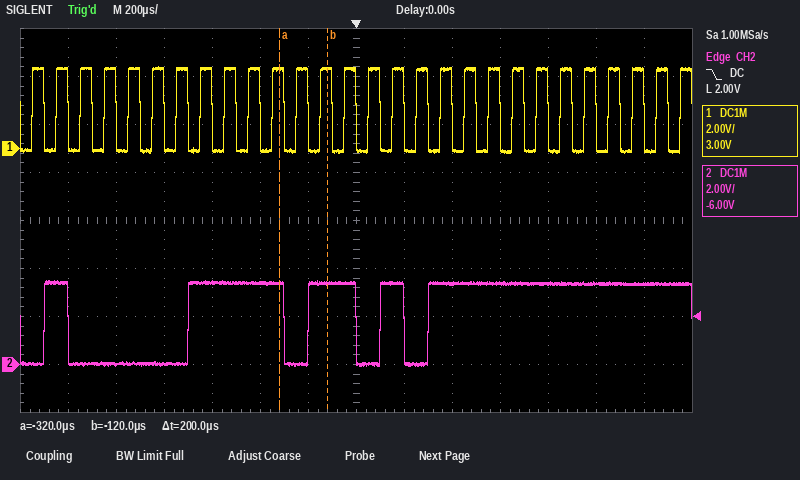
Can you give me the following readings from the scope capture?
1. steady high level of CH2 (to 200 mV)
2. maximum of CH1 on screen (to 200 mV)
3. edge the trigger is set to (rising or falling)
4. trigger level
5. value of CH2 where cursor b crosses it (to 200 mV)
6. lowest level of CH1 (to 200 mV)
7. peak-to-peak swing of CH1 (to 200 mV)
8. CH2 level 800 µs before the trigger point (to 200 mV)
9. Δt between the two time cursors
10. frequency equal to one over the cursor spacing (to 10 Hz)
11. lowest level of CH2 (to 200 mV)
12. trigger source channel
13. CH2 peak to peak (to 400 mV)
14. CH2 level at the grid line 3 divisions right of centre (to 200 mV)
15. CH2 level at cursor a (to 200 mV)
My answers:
3.4 V
3.4 V
falling
2.00 V
3.4 V
-200 mV
3.6 V
0.0 V
200 µs
5.00 kHz
0.0 V
CH2
3.6 V
3.4 V
3.4 V
